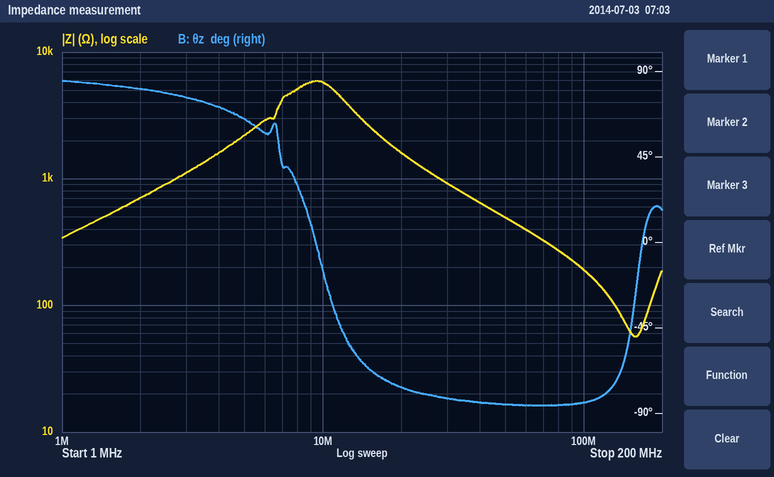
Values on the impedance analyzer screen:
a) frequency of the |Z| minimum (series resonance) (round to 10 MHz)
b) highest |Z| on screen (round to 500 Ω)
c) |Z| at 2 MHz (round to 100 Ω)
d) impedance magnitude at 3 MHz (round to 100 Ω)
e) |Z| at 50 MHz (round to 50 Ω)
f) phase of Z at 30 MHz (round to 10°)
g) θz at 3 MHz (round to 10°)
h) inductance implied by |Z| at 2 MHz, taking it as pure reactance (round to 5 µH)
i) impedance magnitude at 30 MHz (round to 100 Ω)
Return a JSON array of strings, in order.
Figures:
["160 MHz", "6.0 kΩ", "700 Ω", "1.1 kΩ", "500 Ω", "-80°", "80°", "55 µH", "900 Ω"]
